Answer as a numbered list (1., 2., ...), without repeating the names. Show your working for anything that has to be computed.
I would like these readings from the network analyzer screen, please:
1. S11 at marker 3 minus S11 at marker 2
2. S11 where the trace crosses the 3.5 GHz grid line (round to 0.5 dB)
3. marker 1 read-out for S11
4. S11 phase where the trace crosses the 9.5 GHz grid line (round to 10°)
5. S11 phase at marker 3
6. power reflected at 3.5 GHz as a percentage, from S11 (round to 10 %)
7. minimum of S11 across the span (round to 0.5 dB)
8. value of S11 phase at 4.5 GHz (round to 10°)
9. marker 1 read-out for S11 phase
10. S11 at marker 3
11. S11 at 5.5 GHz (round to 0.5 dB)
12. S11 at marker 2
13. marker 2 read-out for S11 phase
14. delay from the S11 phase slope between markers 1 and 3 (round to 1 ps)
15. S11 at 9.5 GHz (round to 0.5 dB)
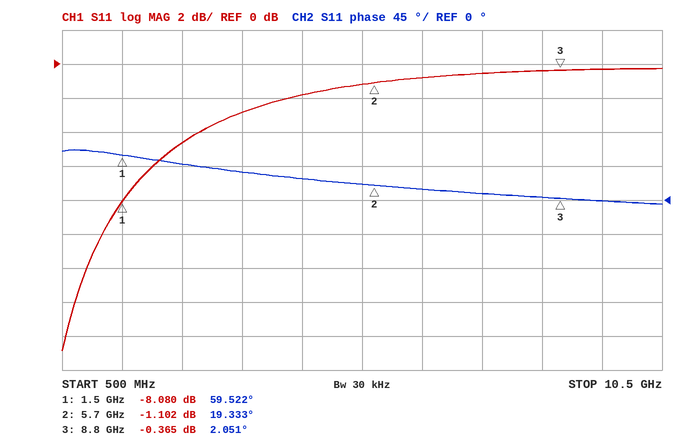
1. -0.365 − (-1.102) = 0.737 dB
2. -3.0 dB
3. -8.080 dB
4. 0°
5. 2.051°
6. 10^(-3/10) ≈ 50 %
7. -17.0 dB
8. 30°
9. 59.522°
10. -0.365 dB
11. -1.0 dB
12. -1.102 dB
13. 19.333°
14. −(2.051° − (59.522°))/(360° × 7.3 GHz) ≈ 22 ps
15. -0.5 dB
